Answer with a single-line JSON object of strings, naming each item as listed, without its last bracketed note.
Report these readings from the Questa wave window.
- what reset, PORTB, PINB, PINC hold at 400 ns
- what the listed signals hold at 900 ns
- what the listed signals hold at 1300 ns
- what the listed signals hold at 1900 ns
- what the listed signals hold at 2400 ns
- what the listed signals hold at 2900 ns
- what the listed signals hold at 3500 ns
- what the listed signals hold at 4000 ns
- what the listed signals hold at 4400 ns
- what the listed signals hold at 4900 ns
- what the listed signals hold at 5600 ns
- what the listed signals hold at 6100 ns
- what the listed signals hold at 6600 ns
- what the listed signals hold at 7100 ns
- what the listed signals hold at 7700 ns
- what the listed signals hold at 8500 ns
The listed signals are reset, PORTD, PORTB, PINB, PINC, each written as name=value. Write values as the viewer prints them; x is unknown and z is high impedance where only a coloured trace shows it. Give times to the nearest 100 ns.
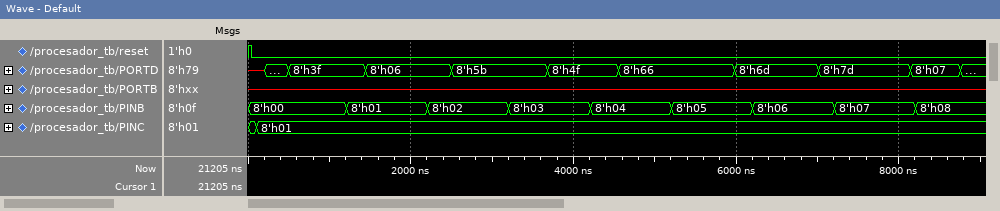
{"what reset, PORTB, PINB, PINC hold at 400 ns": "reset=0, PORTB=x, PINB=8'h00, PINC=8'h01", "what the listed signals hold at 900 ns": "reset=0, PORTD=8'h3f, PORTB=x, PINB=8'h00, PINC=8'h01", "what the listed signals hold at 1300 ns": "reset=0, PORTD=8'h3f, PORTB=x, PINB=8'h01, PINC=8'h01", "what the listed signals hold at 1900 ns": "reset=0, PORTD=8'h06, PORTB=x, PINB=8'h01, PINC=8'h01", "what the listed signals hold at 2400 ns": "reset=0, PORTD=8'h06, PORTB=x, PINB=8'h02, PINC=8'h01", "what the listed signals hold at 2900 ns": "reset=0, PORTD=8'h5b, PORTB=x, PINB=8'h02, PINC=8'h01", "what the listed signals hold at 3500 ns": "reset=0, PORTD=8'h5b, PORTB=x, PINB=8'h03, PINC=8'h01", "what the listed signals hold at 4000 ns": "reset=0, PORTD=8'h4f, PORTB=x, PINB=8'h03, PINC=8'h01", "what the listed signals hold at 4400 ns": "reset=0, PORTD=8'h4f, PORTB=x, PINB=8'h04, PINC=8'h01", "what the listed signals hold at 4900 ns": "reset=0, PORTD=8'h66, PORTB=x, PINB=8'h04, PINC=8'h01", "what the listed signals hold at 5600 ns": "reset=0, PORTD=8'h66, PORTB=x, PINB=8'h05, PINC=8'h01", "what the listed signals hold at 6100 ns": "reset=0, PORTD=8'h6d, PORTB=x, PINB=8'h05, PINC=8'h01", "what the listed signals hold at 6600 ns": "reset=0, PORTD=8'h6d, PORTB=x, PINB=8'h06, PINC=8'h01", "what the listed signals hold at 7100 ns": "reset=0, PORTD=8'h7d, PORTB=x, PINB=8'h06, PINC=8'h01", "what the listed signals hold at 7700 ns": "reset=0, PORTD=8'h7d, PORTB=x, PINB=8'h07, PINC=8'h01", "what the listed signals hold at 8500 ns": "reset=0, PORTD=8'h07, PORTB=x, PINB=8'h08, PINC=8'h01"}
